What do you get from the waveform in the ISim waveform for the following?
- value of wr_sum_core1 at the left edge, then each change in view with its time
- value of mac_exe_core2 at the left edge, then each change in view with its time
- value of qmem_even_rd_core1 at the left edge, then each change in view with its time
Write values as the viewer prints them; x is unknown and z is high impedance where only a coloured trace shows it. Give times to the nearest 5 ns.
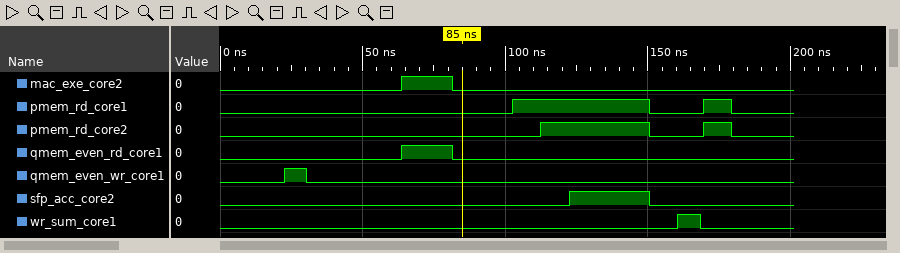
0, 1 at 160 ns, 0 at 170 ns
0, 1 at 65 ns, 0 at 80 ns
0, 1 at 65 ns, 0 at 80 ns
